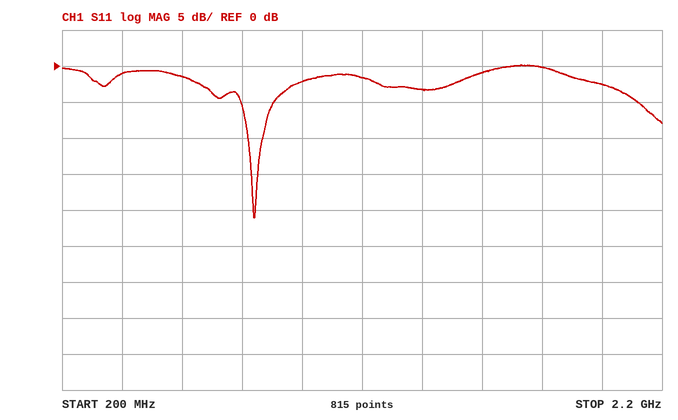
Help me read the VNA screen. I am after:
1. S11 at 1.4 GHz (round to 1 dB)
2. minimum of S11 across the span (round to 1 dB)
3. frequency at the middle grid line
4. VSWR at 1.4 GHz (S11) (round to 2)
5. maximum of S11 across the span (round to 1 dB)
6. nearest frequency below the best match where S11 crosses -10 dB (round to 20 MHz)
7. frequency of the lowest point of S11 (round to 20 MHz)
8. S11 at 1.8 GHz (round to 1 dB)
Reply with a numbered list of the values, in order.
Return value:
1. -3 dB
2. -21 dB
3. 1.2 GHz
4. 6
5. 0 dB
6. 820 MHz
7. 840 MHz
8. 0 dB
